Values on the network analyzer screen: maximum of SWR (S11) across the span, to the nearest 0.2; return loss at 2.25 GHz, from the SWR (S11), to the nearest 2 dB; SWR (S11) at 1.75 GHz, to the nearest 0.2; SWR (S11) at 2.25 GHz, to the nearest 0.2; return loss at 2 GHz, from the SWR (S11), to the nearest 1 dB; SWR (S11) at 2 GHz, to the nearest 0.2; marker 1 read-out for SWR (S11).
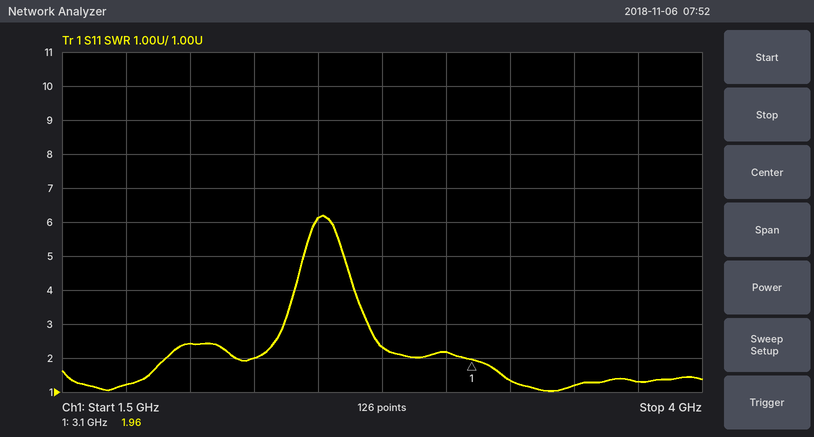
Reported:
6.2
10 dB
1.2
2.0
8 dB
2.4
1.96
